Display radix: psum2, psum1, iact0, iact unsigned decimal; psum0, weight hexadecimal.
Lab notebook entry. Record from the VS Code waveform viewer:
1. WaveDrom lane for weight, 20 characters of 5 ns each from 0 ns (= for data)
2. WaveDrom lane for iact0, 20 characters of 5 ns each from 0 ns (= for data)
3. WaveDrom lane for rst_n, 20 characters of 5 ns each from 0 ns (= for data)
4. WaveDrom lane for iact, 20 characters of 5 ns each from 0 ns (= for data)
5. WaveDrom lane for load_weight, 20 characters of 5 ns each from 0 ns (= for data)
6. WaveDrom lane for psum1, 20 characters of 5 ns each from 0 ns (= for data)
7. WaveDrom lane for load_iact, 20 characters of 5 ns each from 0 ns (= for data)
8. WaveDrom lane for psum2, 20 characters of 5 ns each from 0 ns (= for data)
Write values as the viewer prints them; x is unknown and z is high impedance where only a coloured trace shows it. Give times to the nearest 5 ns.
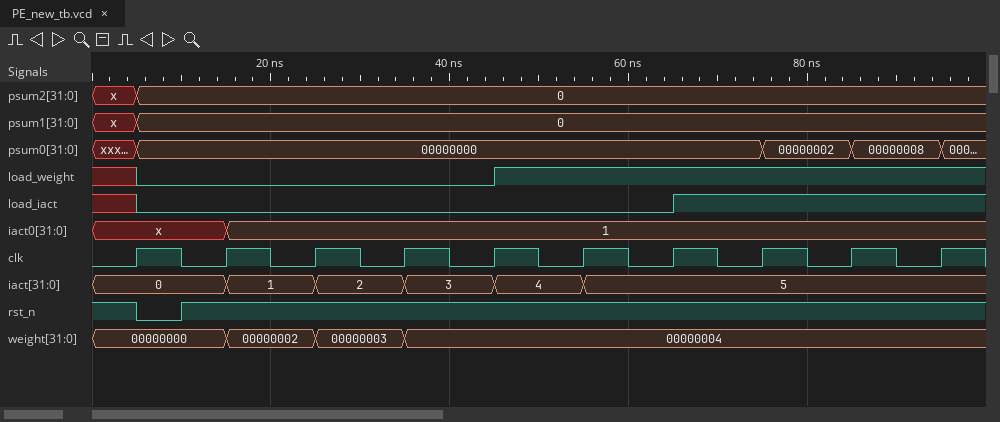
{name: 'weight', wave: '=..=.=.=............', data: '00000000 00000002 00000003 00000004'}
{name: 'iact0', wave: 'x..=................', data: '1'}
{name: 'rst_n', wave: '101.................'}
{name: 'iact', wave: '=..=.=.=.=.=........', data: '0 1 2 3 4 5'}
{name: 'load_weight', wave: 'x0.......1..........'}
{name: 'psum1', wave: 'x=..................', data: '0'}
{name: 'load_iact', wave: 'x0...........1......'}
{name: 'psum2', wave: 'x=..................', data: '0'}
